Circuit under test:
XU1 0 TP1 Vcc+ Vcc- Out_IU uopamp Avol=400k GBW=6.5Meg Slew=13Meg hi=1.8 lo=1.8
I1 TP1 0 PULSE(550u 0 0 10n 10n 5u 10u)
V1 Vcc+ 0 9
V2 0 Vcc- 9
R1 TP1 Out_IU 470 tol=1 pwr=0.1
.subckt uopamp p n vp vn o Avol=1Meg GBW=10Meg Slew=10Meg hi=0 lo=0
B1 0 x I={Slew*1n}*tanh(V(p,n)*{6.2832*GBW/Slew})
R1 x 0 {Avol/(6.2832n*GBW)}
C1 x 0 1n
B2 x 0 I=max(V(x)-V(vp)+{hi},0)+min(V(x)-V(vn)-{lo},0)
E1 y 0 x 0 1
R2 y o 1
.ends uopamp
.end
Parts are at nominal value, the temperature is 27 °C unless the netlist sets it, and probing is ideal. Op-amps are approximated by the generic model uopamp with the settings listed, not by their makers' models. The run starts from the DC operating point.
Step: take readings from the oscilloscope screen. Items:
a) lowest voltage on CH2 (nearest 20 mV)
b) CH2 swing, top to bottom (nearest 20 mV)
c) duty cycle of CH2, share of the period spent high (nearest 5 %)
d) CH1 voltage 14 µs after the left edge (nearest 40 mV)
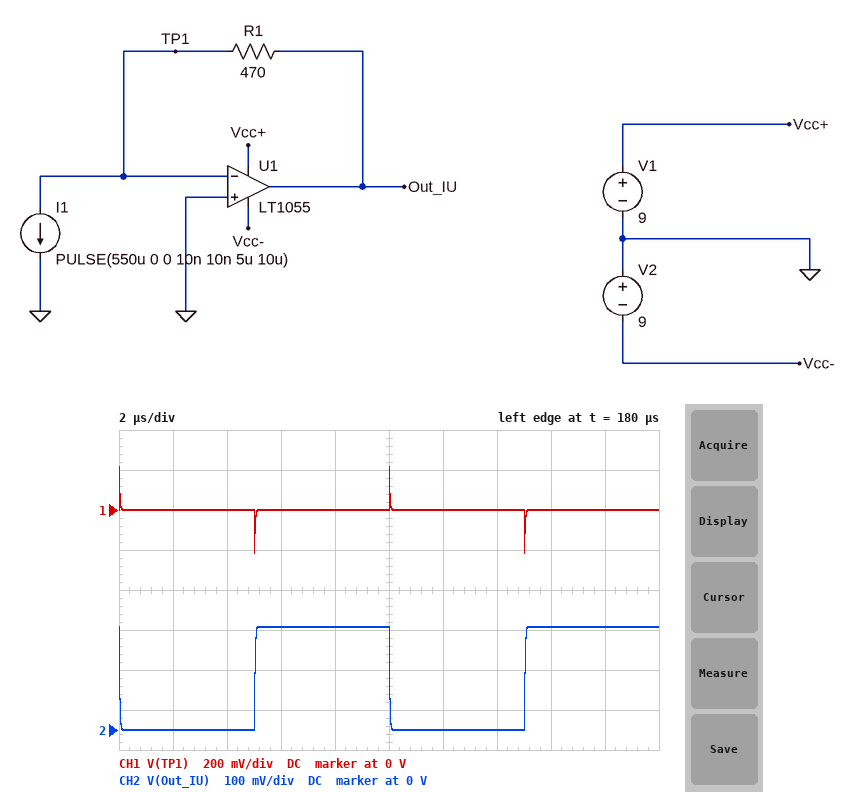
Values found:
0 V
260 mV
50 %
0 V
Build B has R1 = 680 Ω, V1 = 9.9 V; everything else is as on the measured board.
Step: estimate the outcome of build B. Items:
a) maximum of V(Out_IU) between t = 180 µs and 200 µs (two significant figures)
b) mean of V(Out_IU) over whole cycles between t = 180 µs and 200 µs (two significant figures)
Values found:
370 mV
190 mV
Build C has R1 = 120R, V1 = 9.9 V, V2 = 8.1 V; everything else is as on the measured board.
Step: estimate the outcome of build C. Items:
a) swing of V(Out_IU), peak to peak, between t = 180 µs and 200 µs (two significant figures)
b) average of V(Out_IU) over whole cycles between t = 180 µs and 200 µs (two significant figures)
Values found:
66 mV
33 mV
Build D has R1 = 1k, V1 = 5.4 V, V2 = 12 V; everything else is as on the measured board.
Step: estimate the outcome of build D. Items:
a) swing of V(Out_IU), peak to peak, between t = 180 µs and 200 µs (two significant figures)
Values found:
550 mV
